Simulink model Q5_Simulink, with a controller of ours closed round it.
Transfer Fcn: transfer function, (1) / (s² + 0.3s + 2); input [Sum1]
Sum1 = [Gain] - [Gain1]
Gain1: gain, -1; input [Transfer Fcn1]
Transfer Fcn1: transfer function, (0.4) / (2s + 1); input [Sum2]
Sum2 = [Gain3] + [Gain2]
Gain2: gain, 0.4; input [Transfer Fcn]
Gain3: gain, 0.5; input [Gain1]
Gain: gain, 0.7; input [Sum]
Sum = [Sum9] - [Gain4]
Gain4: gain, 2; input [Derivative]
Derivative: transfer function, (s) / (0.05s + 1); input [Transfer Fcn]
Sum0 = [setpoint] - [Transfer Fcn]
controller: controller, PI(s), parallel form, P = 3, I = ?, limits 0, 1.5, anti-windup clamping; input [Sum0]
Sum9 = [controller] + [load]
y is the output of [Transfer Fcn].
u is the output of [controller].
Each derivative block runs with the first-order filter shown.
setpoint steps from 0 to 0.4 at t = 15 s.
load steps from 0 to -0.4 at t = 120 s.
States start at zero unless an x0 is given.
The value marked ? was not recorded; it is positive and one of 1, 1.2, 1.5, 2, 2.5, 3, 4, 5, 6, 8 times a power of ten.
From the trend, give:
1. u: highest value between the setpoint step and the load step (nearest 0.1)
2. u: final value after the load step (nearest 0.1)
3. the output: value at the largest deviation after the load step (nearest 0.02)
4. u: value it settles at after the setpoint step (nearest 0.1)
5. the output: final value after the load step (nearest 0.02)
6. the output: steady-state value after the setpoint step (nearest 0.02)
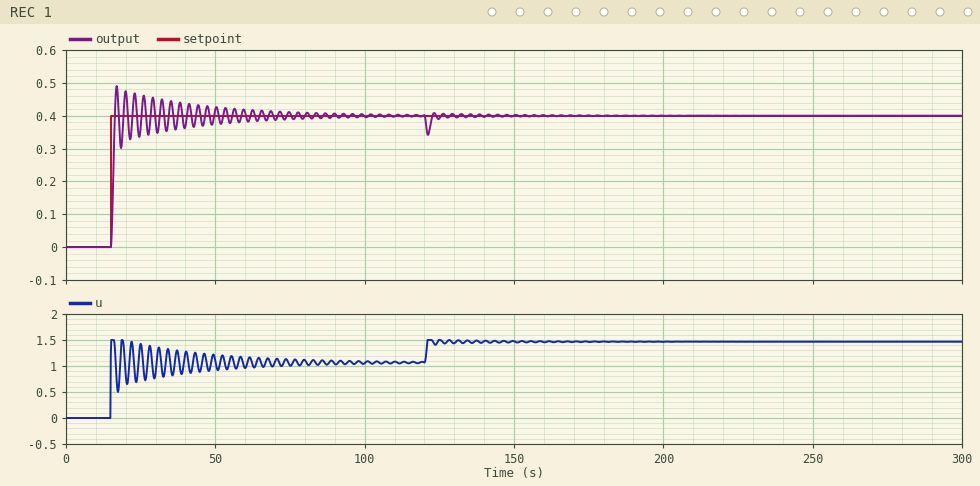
1.5
1.5
0.34
1.1
0.40
0.40
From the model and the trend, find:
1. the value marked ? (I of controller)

10
